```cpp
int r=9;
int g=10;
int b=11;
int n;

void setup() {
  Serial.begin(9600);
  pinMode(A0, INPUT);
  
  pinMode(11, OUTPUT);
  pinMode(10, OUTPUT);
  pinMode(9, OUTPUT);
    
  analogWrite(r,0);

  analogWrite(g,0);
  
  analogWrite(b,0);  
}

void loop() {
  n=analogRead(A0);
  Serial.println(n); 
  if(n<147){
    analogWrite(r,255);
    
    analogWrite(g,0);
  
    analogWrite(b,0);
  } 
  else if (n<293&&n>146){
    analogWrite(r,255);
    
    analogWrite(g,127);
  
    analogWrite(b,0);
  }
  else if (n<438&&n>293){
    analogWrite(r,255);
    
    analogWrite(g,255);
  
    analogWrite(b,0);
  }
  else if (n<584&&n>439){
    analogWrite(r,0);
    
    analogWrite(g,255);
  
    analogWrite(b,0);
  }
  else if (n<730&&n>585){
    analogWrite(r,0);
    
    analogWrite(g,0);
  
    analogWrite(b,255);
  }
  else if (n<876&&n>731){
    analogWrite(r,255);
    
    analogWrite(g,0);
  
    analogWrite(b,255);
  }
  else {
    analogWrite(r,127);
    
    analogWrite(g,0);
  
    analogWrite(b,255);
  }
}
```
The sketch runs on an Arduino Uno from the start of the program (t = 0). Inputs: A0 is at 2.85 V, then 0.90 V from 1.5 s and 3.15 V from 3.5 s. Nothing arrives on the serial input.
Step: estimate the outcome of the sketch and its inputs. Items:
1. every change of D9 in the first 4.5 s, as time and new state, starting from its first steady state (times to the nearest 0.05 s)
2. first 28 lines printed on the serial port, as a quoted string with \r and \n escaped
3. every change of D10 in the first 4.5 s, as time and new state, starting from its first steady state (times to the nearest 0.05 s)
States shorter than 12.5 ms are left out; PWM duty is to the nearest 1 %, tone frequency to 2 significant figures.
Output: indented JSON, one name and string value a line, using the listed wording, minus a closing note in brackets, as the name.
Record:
{
  "every change of D9 in the first 4.5 s, as time and new state, starting from its first steady state": "0 s low; 1.5 s high; 3.5 s low",
  "first 28 lines printed on the serial port, as a quoted string with \\r and \\n escaped": "\"583\\r\\n583\\r\\n583\\r\\n583\\r\\n583\\r\\n583\\r\\n583\\r\\n583\\r\\n583\\r\\n583\\r\\n583\\r\\n583\\r\\n583\\r\\n583\\r\\n583\\r\\n583\\r\\n583\\r\\n583\\r\\n583\\r\\n583\\r\\n583\\r\\n583\\r\\n583\\r\\n583\\r\\n583\\r\\n583\\r\\n583\\r\\n583\\r\\n\"",
  "every change of D10 in the first 4.5 s, as time and new state, starting from its first steady state": "0 s high; 1.5 s PWM 50 %; 3.5 s low"
}
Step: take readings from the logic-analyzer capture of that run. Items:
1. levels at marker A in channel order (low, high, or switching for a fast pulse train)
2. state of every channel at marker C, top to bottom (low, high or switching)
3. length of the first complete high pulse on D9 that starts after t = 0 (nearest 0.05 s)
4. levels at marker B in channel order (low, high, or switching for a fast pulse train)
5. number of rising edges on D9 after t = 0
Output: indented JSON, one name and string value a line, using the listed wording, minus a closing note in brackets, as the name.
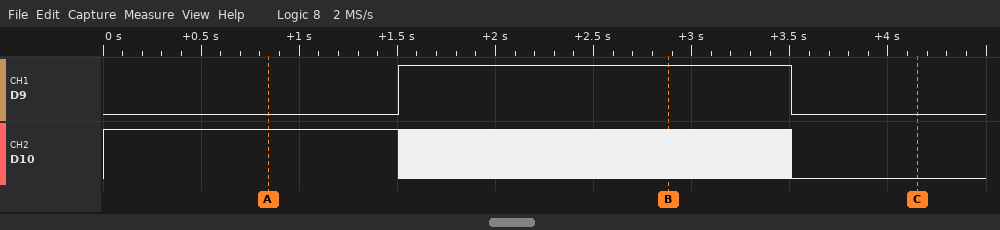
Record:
{
  "levels at marker A in channel order": "D9 low, D10 high",
  "state of every channel at marker C, top to bottom": "D9 low, D10 low",
  "length of the first complete high pulse on D9 that starts after t = 0": "2.00 s",
  "levels at marker B in channel order": "D9 high, D10 switching",
  "number of rising edges on D9 after t = 0": "1"
}
